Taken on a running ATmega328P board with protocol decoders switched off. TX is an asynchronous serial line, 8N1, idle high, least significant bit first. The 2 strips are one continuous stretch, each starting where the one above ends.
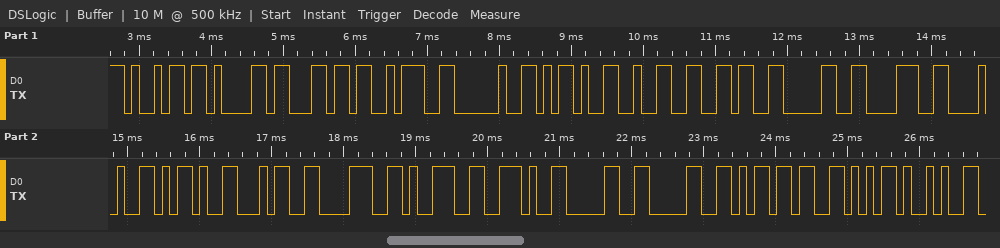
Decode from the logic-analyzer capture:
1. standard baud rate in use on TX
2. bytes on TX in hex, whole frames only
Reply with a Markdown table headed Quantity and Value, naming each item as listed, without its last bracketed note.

| Quantity | Value |
|---|---|
| standard baud rate in use on TX | 9600 baud |
| bytes on TX in hex, whole frames only | 69 61 6C 3A 20 2D 32 36 30 38 28 2D 34 38 39 2E 30 30 6D 56 29 |
